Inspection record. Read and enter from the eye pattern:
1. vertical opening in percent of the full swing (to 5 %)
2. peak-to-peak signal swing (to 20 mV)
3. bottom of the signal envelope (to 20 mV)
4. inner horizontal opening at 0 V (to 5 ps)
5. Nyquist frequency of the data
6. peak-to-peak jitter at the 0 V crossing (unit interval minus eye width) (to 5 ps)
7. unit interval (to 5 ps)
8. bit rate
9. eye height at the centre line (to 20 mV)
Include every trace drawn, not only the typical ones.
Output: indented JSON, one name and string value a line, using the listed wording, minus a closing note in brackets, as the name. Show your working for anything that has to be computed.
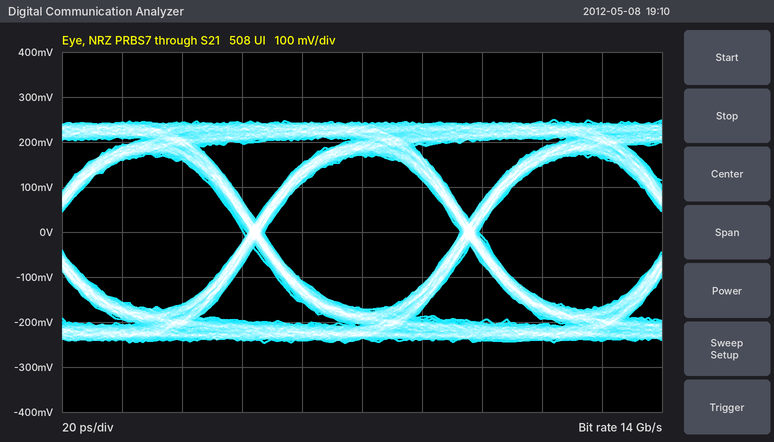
{
  "vertical opening in percent of the full swing": "340 mV / 500 mV ≈ 68.0 %, so 70 % to the nearest 5 %",
  "peak-to-peak signal swing": "500 mV",
  "bottom of the signal envelope": "-240 mV",
  "inner horizontal opening at 0 V": "65 ps",
  "Nyquist frequency of the data": "7 GHz",
  "peak-to-peak jitter at the 0 V crossing (unit interval minus eye width)": "5 ps",
  "unit interval": "70 ps",
  "bit rate": "14 Gb/s",
  "eye height at the centre line": "340 mV"
}
